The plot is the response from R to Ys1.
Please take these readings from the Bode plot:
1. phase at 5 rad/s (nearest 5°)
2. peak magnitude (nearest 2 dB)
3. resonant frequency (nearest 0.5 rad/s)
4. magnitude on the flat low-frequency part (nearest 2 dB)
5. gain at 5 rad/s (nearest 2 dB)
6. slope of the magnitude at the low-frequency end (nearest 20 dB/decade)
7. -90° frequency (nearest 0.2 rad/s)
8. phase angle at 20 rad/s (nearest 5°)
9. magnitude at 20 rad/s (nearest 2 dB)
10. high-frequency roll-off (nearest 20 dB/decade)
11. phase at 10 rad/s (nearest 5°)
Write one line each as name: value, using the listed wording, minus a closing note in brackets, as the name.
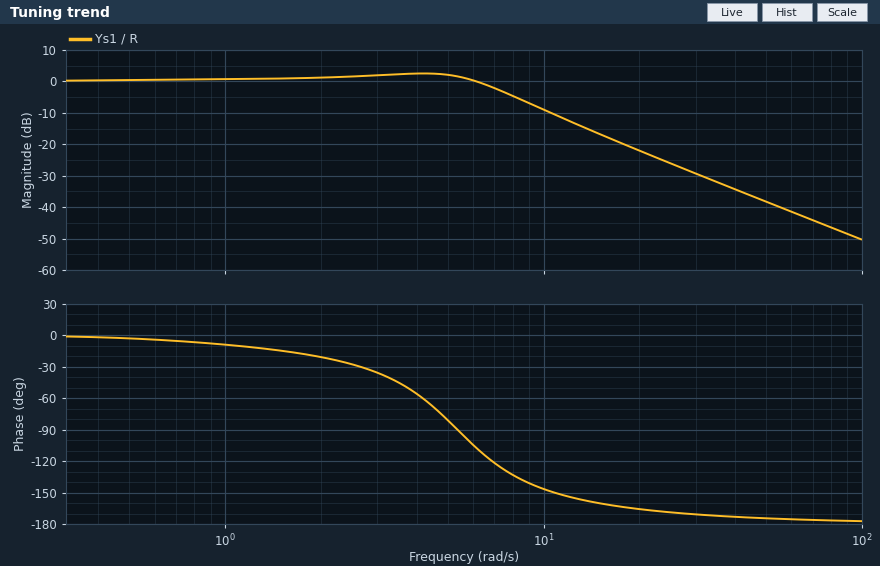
phase at 5 rad/s: -80°
peak magnitude: 2 dB
resonant frequency: 4.0 rad/s
magnitude on the flat low-frequency part: 0 dB
gain at 5 rad/s: 2 dB
slope of the magnitude at the low-frequency end: 0 dB/decade
-90° frequency: 5.4 rad/s
phase angle at 20 rad/s: -165°
magnitude at 20 rad/s: -22 dB
high-frequency roll-off: -40 dB/decade
phase at 10 rad/s: -145°
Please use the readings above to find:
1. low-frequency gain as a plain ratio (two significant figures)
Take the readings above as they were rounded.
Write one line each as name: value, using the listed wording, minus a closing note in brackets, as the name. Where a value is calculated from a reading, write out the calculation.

low-frequency gain as a plain ratio: 10^(0 / 20) = 1.0
